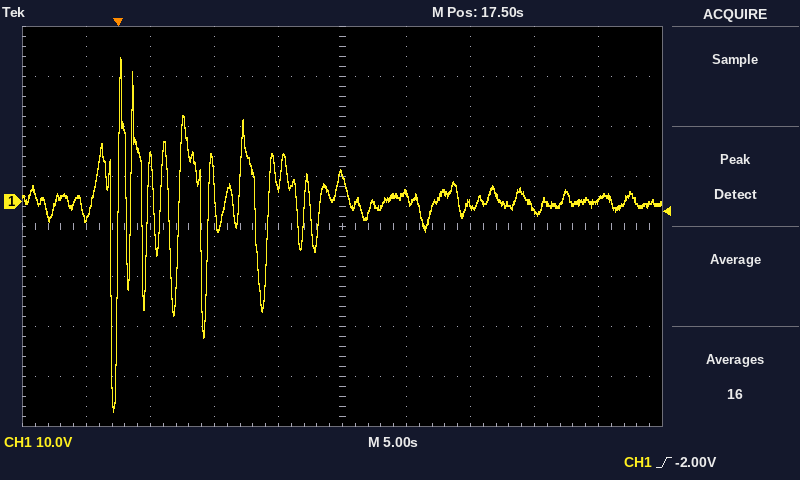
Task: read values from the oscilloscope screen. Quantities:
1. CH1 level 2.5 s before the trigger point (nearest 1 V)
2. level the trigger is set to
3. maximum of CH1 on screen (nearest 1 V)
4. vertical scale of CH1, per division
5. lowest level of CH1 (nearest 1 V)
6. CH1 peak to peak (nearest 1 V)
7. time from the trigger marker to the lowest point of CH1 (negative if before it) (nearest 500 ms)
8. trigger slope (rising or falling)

-3 V
-2.00 V
29 V
10 V
-42 V
71 V
-500 ms
rising
